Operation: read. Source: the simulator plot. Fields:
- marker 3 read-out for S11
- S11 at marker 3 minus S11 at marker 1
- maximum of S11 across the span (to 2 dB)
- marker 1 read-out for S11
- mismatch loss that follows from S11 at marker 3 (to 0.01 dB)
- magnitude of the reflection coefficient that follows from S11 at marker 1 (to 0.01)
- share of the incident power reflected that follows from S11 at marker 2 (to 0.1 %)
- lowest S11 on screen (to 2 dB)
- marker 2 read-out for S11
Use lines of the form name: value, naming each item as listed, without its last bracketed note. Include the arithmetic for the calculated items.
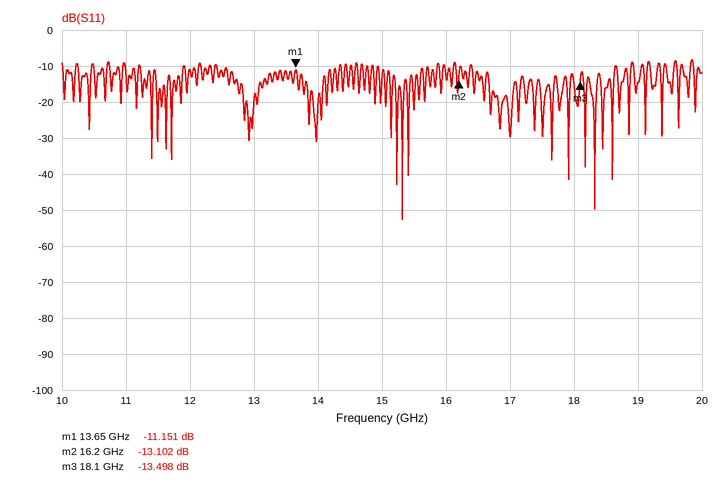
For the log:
marker 3 read-out for S11: -13.498 dB
S11 at marker 3 minus S11 at marker 1: -13.498 − (-11.151) = -2.347 dB
maximum of S11 across the span: -8 dB
marker 1 read-out for S11: -11.151 dB
mismatch loss that follows from S11 at marker 3: −10 log10(1 − 10^(-13.498/10)) ≈ 0.20 dB
magnitude of the reflection coefficient that follows from S11 at marker 1: 10^(-11.151/20) ≈ 0.28
share of the incident power reflected that follows from S11 at marker 2: 10^(-13.102/10) ≈ 4.9 %
lowest S11 on screen: -52 dB
marker 2 read-out for S11: -13.102 dB
